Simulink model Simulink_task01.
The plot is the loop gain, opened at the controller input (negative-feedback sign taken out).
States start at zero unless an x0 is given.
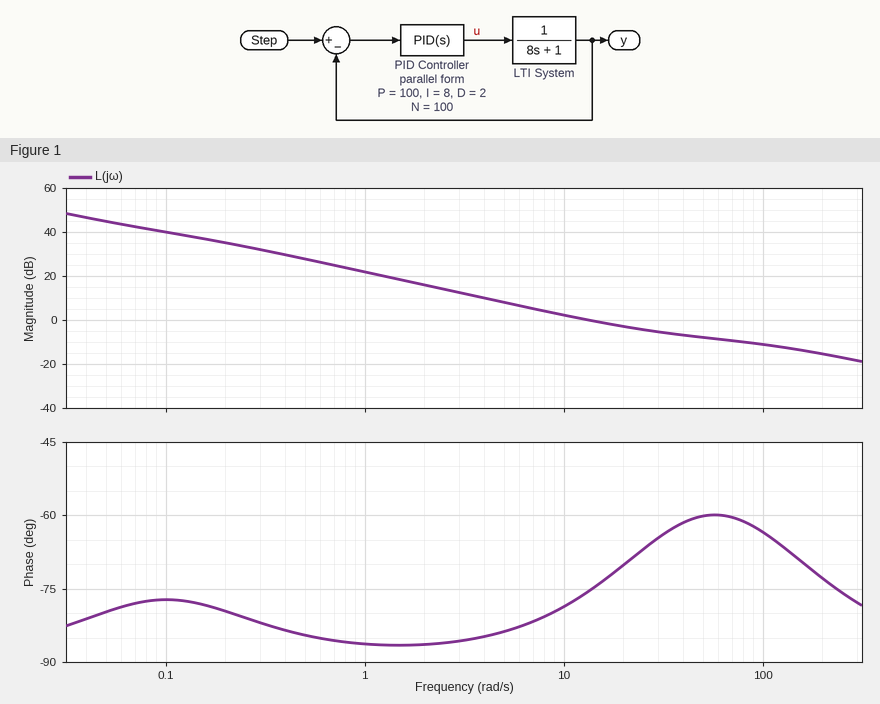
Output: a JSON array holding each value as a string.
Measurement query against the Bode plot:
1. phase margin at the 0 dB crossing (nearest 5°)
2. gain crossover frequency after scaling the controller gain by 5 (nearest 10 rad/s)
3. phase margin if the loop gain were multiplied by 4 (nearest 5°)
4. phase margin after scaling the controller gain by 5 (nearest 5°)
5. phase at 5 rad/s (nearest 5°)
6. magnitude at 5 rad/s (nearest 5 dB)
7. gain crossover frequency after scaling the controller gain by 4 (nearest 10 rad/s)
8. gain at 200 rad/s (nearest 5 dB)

["105°", "160 rad/s", "115°", "110°", "-85°", "10 dB", "120 rad/s", "-15 dB"]
